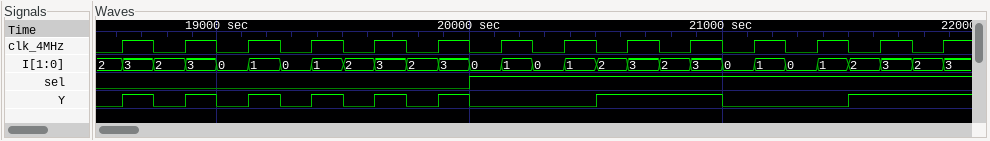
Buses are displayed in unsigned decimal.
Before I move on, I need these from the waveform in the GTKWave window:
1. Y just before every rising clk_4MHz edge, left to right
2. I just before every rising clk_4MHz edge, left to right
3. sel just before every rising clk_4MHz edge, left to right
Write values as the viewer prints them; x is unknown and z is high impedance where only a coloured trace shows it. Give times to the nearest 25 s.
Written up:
0 0 0 0 0 0 0 0 1 1 0 0 1 1
2, 2, 0, 0, 2, 2, 0, 0, 2, 2, 0, 0, 2, 2
0 0 0 0 0 0 1 1 1 1 1 1 1 1
